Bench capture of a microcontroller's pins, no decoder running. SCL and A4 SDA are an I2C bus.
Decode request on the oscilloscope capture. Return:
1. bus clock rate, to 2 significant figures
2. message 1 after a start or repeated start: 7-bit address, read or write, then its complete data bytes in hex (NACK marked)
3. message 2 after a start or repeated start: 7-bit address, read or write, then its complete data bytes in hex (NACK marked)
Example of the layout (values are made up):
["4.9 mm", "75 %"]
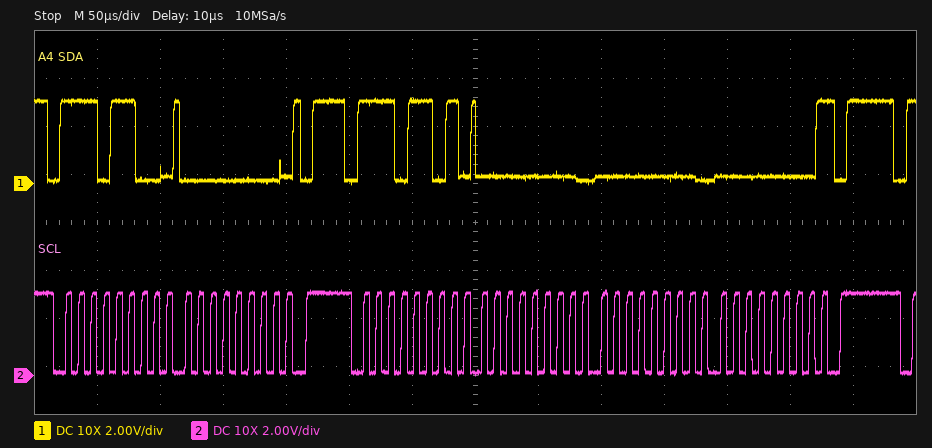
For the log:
["100 kHz", "0x76 write: 00", "0x76 read: 00 00 00 NACK"]
